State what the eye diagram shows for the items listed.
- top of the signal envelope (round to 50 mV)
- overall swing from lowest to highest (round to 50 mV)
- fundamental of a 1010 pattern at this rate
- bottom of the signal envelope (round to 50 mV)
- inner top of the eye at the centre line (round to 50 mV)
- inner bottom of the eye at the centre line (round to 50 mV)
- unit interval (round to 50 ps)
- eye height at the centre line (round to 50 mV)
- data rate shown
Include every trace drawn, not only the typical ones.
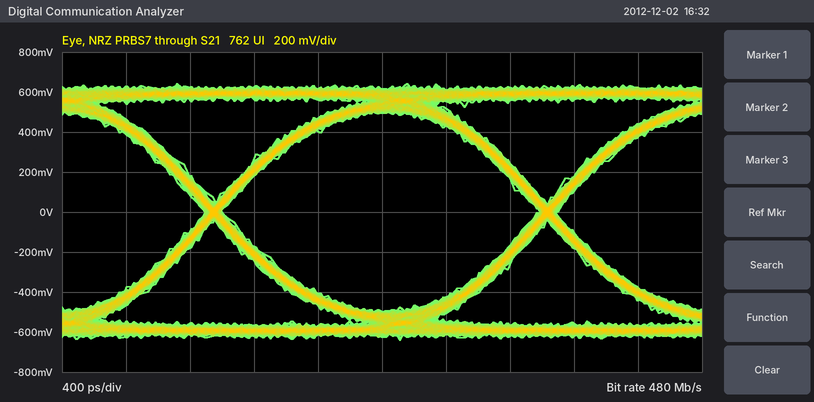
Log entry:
650 mV
1.30 V
240 MHz
-650 mV
500 mV
-500 mV
2.10 ns
1.00 V
480 Mb/s
